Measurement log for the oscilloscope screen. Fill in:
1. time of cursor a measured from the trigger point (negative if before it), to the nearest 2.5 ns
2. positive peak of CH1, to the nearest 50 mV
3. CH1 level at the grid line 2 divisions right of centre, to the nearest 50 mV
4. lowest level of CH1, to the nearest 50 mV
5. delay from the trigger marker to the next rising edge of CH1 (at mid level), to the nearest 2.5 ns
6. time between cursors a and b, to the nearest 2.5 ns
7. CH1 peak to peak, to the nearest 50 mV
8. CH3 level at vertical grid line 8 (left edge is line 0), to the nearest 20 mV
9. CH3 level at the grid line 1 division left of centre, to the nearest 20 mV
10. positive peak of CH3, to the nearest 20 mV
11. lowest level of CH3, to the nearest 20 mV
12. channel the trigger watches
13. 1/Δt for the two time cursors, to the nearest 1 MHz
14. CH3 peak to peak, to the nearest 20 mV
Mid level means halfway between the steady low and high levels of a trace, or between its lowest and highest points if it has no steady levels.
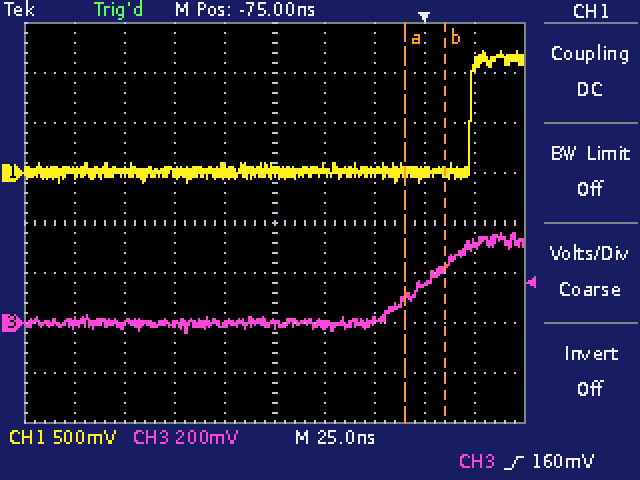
-10.0 ns
1.20 V
0 mV
-100 mV
22.5 ns
20.0 ns
1.30 V
160 mV
0 mV
360 mV
-40 mV
CH3
50 MHz
400 mV
